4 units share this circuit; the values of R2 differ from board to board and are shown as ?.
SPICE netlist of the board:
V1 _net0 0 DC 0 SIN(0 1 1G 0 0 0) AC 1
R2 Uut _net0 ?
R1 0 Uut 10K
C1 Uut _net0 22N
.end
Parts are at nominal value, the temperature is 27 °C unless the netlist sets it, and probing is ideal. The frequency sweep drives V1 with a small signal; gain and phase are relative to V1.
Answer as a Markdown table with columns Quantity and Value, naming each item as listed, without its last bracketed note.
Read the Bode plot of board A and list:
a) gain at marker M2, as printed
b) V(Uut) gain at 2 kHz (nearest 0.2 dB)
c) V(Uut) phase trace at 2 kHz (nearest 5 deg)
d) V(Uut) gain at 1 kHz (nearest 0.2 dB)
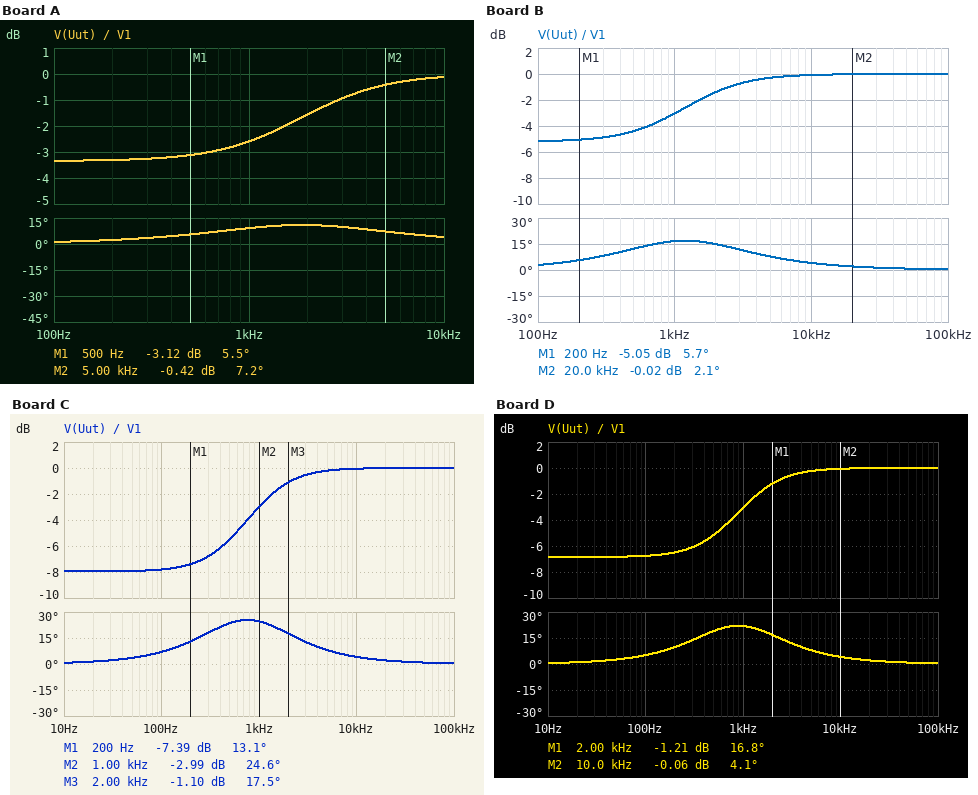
| Quantity | Value |
|---|---|
| gain at marker M2, as printed | -0.42 dB |
| V(Uut) gain at 2 kHz | -1.6 dB |
| V(Uut) phase trace at 2 kHz | 10 deg |
| V(Uut) gain at 1 kHz | -2.6 dB |
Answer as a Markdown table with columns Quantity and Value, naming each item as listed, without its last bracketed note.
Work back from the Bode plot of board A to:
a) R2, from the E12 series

| Quantity | Value |
|---|---|
| R2, from the E12 series | 4.7 kΩ |
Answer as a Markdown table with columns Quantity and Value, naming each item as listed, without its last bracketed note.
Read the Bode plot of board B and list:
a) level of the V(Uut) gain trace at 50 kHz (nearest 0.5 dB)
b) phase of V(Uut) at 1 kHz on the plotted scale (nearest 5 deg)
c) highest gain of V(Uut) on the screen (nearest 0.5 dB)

| Quantity | Value |
|---|---|
| level of the V(Uut) gain trace at 50 kHz | 0 dB |
| phase of V(Uut) at 1 kHz on the plotted scale | 15 deg |
| highest gain of V(Uut) on the screen | 0 dB |
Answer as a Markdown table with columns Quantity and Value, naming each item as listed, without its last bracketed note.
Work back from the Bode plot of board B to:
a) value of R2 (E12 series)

| Quantity | Value |
|---|---|
| value of R2 | 8.2 kΩ |
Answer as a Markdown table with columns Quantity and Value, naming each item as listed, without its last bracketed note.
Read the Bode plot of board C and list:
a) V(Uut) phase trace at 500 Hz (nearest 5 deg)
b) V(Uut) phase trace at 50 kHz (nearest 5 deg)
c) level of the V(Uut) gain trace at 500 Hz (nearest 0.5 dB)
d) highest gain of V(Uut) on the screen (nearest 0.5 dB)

| Quantity | Value |
|---|---|
| V(Uut) phase trace at 500 Hz | 25 deg |
| V(Uut) phase trace at 50 kHz | 0 deg |
| level of the V(Uut) gain trace at 500 Hz | -5.5 dB |
| highest gain of V(Uut) on the screen | 0 dB |
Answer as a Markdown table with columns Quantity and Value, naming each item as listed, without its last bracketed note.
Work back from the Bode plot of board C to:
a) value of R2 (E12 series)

| Quantity | Value |
|---|---|
| value of R2 | 15 kΩ |
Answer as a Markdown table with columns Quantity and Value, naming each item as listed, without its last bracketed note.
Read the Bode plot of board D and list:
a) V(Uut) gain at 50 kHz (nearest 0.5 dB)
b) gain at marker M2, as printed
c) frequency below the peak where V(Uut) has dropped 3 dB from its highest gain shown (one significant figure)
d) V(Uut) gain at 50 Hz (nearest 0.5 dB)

| Quantity | Value |
|---|---|
| V(Uut) gain at 50 kHz | 0 dB |
| gain at marker M2, as printed | -0.06 dB |
| frequency below the peak where V(Uut) has dropped 3 dB from its highest gain shown | 1 kHz |
| V(Uut) gain at 50 Hz | -7.0 dB |
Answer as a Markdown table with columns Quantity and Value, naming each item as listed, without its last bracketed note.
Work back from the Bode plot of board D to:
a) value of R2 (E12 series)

| Quantity | Value |
|---|---|
| value of R2 | 12 kΩ |
